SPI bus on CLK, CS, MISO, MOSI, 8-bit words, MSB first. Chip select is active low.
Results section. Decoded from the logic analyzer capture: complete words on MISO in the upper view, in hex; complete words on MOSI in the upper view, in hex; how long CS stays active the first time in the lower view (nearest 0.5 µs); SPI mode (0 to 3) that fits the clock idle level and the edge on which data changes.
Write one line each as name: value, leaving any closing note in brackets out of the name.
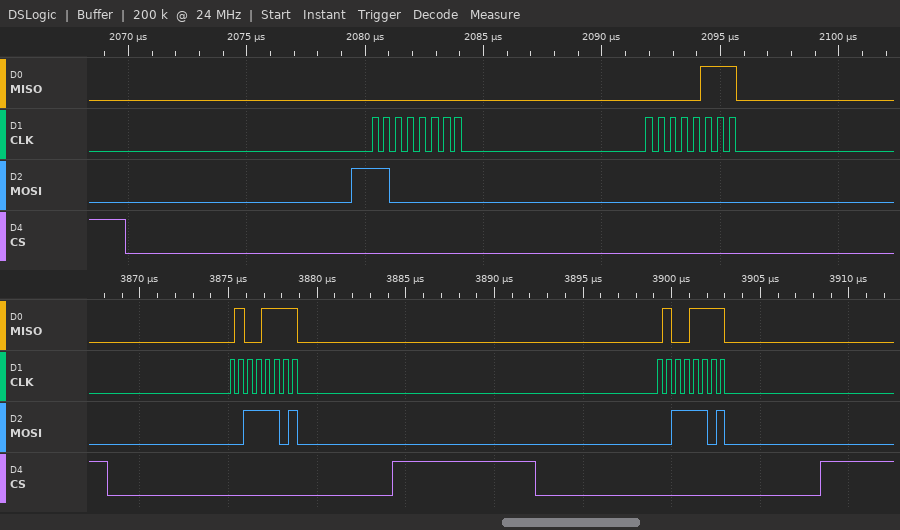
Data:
complete words on MISO in the upper view, in hex: 00, 07
complete words on MOSI in the upper view, in hex: C0, 00
how long CS stays active the first time in the lower view: 16 µs
SPI mode (0 to 3) that fits the clock idle level and the edge on which data changes: 0
